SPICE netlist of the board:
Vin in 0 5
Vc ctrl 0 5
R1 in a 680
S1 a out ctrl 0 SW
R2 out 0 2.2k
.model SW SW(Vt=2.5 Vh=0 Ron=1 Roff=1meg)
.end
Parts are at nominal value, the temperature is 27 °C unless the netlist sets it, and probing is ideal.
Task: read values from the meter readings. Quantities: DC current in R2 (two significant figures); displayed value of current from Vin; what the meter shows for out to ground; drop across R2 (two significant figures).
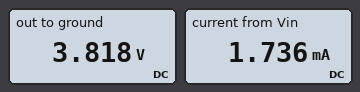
1.7 mA
1.736 mA
3.818 V
3.8 V
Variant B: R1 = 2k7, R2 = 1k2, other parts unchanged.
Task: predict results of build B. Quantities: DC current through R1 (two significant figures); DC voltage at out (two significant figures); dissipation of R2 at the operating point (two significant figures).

1.3 mA
1.5 V
2.0 mW
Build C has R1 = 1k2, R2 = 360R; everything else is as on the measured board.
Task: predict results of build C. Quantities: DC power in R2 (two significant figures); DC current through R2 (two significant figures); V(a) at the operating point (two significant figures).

3.7 mW
3.2 mA
1.2 V
